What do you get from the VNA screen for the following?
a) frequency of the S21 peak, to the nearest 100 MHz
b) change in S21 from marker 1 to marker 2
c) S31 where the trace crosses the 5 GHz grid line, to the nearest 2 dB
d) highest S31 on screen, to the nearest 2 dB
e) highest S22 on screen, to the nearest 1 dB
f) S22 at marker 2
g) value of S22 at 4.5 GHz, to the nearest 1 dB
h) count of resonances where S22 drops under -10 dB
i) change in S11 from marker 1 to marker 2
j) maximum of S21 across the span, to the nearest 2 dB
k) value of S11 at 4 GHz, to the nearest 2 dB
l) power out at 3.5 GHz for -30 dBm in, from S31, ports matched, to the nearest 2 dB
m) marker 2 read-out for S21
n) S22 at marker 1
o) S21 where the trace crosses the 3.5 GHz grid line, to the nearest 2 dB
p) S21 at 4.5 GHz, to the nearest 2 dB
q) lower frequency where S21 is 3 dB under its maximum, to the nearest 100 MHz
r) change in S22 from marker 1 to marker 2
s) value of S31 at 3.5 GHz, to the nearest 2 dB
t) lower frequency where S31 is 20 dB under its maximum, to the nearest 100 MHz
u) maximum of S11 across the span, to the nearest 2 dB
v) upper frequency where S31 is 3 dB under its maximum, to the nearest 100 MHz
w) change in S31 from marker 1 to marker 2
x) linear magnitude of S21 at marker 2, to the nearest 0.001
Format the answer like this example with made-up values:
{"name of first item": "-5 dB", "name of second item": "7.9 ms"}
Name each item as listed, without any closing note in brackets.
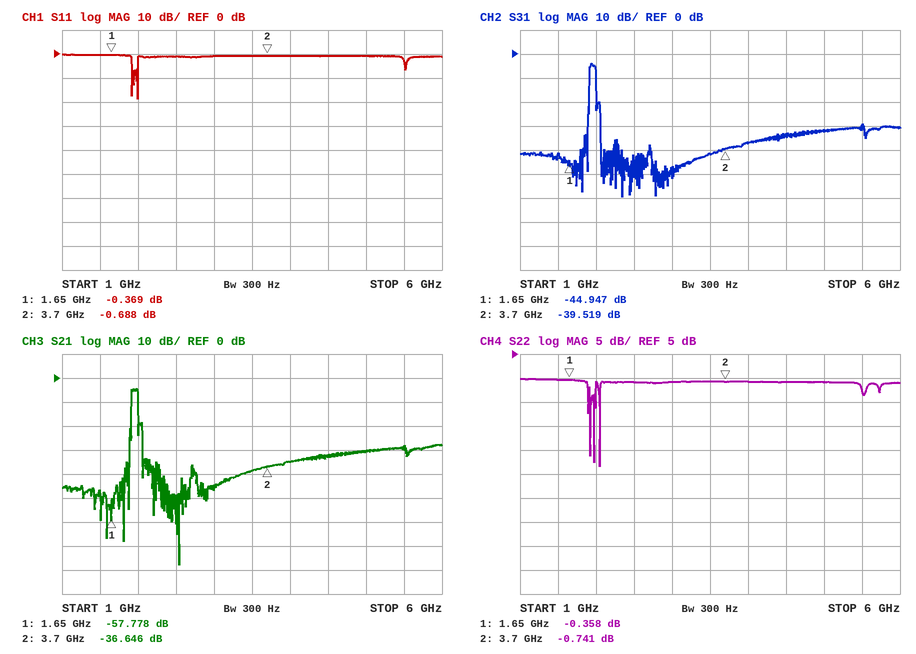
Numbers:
{"frequency of the S21 peak, to the nearest 100 MHz": "2.0 GHz", "change in S21 from marker 1 to marker 2": "21.132 dB", "S31 where the trace crosses the 5 GHz grid line, to the nearest 2 dB": "-32 dB", "highest S31 on screen, to the nearest 2 dB": "-4 dB", "highest S22 on screen, to the nearest 1 dB": "0 dB", "S22 at marker 2": "-0.741 dB", "value of S22 at 4.5 GHz, to the nearest 1 dB": "-1 dB", "count of resonances where S22 drops under -10 dB": "3", "change in S11 from marker 1 to marker 2": "-0.319 dB", "maximum of S21 across the span, to the nearest 2 dB": "-4 dB", "value of S11 at 4 GHz, to the nearest 2 dB": "0 dB", "power out at 3.5 GHz for -30 dBm in, from S31, ports matched, to the nearest 2 dB": "-72 dBm", "marker 2 read-out for S21": "-36.646 dB", "S22 at marker 1": "-0.358 dB", "S21 where the trace crosses the 3.5 GHz grid line, to the nearest 2 dB": "-38 dB", "S21 at 4.5 GHz, to the nearest 2 dB": "-32 dB", "lower frequency where S21 is 3 dB under its maximum, to the nearest 100 MHz": "1.9 GHz", "change in S22 from marker 1 to marker 2": "-0.383 dB", "value of S31 at 3.5 GHz, to the nearest 2 dB": "-42 dB", "lower frequency where S31 is 20 dB under its maximum, to the nearest 100 MHz": "1.9 GHz", "maximum of S11 across the span, to the nearest 2 dB": "0 dB", "upper frequency where S31 is 3 dB under its maximum, to the nearest 100 MHz": "2.0 GHz", "change in S31 from marker 1 to marker 2": "5.428 dB", "linear magnitude of S21 at marker 2, to the nearest 0.001": "0.015"}
